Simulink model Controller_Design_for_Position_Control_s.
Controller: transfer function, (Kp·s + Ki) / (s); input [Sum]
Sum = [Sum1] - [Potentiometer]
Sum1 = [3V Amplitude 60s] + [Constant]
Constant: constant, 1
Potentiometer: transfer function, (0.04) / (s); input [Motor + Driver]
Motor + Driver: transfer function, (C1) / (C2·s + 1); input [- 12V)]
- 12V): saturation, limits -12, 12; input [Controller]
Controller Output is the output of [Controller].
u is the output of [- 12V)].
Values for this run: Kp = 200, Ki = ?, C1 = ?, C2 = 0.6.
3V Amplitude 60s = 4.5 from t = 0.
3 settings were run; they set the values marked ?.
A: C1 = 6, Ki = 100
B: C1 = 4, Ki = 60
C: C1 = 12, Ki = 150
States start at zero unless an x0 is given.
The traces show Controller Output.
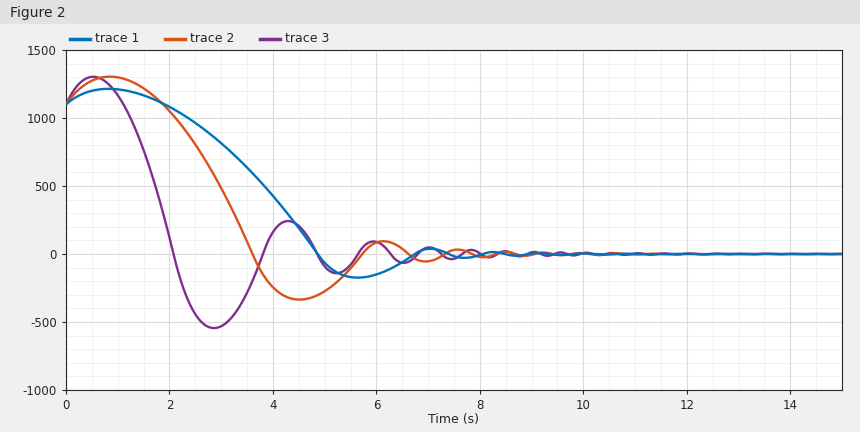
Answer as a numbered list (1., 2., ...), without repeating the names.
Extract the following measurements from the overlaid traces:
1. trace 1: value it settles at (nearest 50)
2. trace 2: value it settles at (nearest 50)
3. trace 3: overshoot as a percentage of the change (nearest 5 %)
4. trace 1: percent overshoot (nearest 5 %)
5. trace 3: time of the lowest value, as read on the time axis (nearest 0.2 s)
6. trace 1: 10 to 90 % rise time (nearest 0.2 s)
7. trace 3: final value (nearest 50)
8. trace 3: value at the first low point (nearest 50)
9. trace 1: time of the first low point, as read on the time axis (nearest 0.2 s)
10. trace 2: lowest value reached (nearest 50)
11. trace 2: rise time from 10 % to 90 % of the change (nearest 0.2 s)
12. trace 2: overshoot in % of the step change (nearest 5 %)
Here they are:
1. 0
2. 0
3. 50 %
4. 15 %
5. 2.8 s
6. 2.2 s
7. 0
8. -550
9. 5.6 s
10. -350
11. 1.4 s
12. 30 %
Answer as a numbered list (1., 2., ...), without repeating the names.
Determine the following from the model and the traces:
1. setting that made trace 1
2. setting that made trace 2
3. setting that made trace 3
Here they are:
1. B
2. A
3. C
